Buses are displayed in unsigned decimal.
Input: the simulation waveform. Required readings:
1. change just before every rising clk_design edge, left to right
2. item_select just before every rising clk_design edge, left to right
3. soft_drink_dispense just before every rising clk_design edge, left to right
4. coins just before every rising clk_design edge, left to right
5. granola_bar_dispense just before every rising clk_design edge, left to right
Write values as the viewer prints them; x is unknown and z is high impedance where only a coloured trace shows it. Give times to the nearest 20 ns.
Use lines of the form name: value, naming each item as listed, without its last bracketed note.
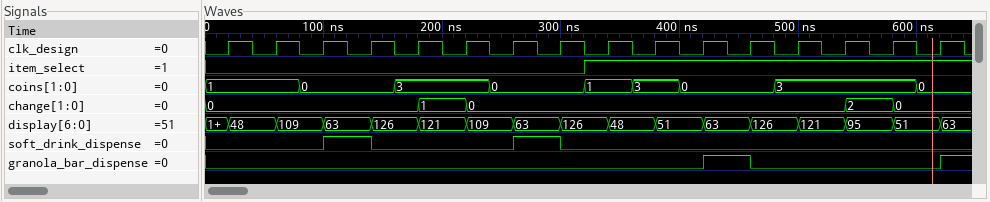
change just before every rising clk_design edge, left to right: 0, 0, 0, 0, 0, 1, 0, 0, 0, 0, 0, 0, 0, 0, 2, 0
item_select just before every rising clk_design edge, left to right: 0 0 0 0 0 0 0 0 1 1 1 1 1 1 1 1
soft_drink_dispense just before every rising clk_design edge, left to right: 0 0 0 1 0 0 0 1 0 0 0 0 0 0 0 0
coins just before every rising clk_design edge, left to right: 1, 1, 0, 0, 3, 3, 0, 0, 1, 3, 0, 0, 3, 3, 3, 0
granola_bar_dispense just before every rising clk_design edge, left to right: 0 0 0 0 0 0 0 0 0 0 0 1 0 0 0 0
